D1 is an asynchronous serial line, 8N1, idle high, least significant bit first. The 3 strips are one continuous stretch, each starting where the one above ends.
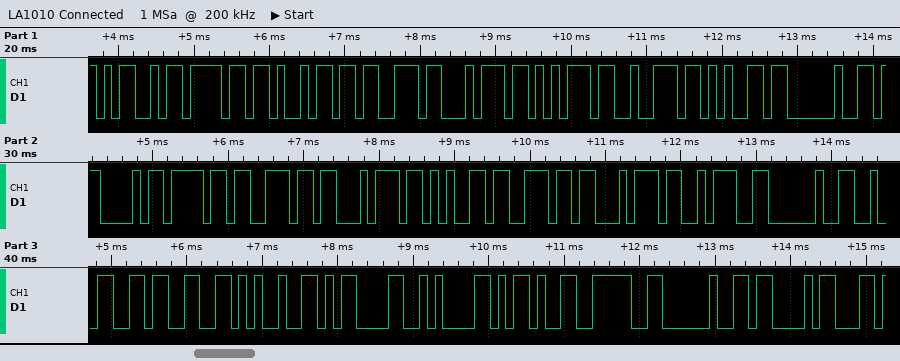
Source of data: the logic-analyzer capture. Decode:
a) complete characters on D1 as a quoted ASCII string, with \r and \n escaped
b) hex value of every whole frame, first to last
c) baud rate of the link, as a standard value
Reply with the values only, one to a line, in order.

"Moisture Content: 23%\r\n-> C"
0x4D 0x6F 0x69 0x73 0x74 0x75 0x72 0x65 0x20 0x43 0x6F 0x6E 0x74 0x65 0x6E 0x74 0x3A 0x20 0x32 0x33 0x25 0x0D 0x0A 0x2D 0x3E 0x20 0x43
9600 baud
